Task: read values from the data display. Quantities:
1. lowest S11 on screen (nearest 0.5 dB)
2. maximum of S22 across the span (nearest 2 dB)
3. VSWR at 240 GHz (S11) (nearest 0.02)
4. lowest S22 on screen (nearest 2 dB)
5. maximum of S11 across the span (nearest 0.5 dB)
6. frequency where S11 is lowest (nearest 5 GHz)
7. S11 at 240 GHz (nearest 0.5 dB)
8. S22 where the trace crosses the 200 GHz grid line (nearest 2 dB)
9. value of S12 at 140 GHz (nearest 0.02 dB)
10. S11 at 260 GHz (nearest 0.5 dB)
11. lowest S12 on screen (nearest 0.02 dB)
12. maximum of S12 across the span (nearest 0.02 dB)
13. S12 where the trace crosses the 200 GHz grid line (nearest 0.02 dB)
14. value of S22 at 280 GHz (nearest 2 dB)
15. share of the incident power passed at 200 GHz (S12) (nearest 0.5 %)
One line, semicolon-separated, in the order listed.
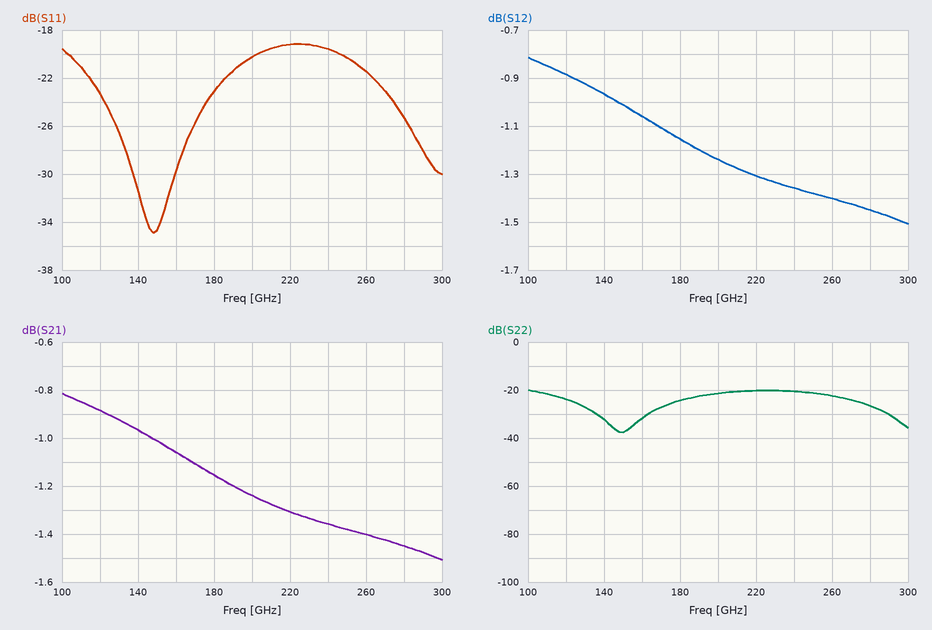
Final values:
-35.0 dB; -20 dB; 1.24; -38 dB; -19.0 dB; 150 GHz; -19.5 dB; -22 dB; -0.96 dB; -21.5 dB; -1.50 dB; -0.82 dB; -1.24 dB; -26 dB; 75.0 %
